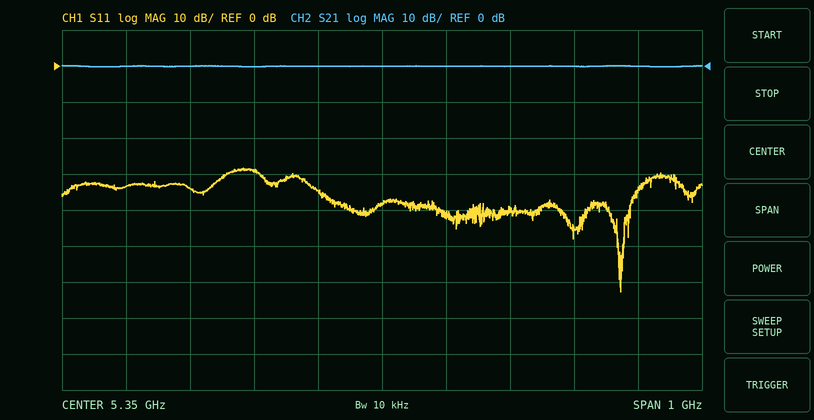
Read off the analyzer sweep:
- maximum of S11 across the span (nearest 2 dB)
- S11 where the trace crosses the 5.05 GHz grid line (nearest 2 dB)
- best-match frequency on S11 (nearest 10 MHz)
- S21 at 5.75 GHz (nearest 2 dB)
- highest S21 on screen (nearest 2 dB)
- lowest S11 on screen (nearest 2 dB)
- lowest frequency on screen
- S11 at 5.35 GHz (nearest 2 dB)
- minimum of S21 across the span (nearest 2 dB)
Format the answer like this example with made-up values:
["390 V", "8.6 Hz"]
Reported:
["-28 dB", "-34 dB", "5.72 GHz", "0 dB", "0 dB", "-62 dB", "4.85 GHz", "-38 dB", "0 dB"]
